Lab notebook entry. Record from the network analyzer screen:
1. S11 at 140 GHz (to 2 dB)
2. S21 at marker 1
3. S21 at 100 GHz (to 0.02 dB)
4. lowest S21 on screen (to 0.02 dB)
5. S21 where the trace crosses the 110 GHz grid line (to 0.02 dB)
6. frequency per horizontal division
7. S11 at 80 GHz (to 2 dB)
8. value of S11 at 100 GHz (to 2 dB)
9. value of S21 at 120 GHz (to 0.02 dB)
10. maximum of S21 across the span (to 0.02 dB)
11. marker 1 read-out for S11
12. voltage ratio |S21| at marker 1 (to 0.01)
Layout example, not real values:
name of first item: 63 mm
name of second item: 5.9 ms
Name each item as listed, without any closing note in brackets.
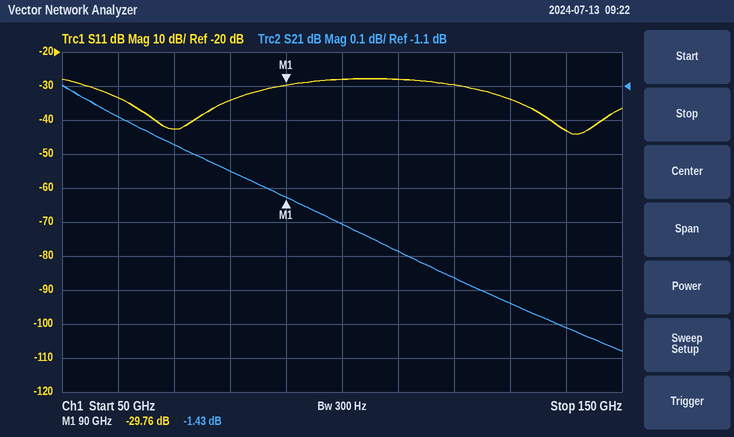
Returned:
S11 at 140 GHz: -44 dB
S21 at marker 1: -1.43 dB
S21 at 100 GHz: -1.50 dB
lowest S21 on screen: -1.88 dB
S21 where the trace crosses the 110 GHz grid line: -1.58 dB
frequency per horizontal division: 10 GHz
S11 at 80 GHz: -34 dB
value of S11 at 100 GHz: -28 dB
value of S21 at 120 GHz: -1.66 dB
maximum of S21 across the span: -1.10 dB
marker 1 read-out for S11: -29.76 dB
voltage ratio |S21| at marker 1: 0.85
